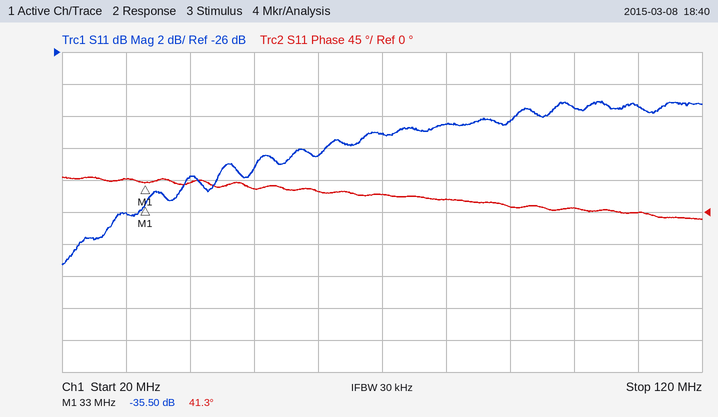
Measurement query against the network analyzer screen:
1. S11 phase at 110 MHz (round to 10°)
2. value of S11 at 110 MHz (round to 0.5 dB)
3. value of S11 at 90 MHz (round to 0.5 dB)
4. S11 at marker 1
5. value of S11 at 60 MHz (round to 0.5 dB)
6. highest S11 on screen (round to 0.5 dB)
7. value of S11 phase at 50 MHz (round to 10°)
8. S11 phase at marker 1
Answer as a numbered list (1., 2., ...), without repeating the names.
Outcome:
1. 0°
2. -29.5 dB
3. -30.5 dB
4. -35.50 dB
5. -32.5 dB
6. -29.0 dB
7. 30°
8. 41.3°
